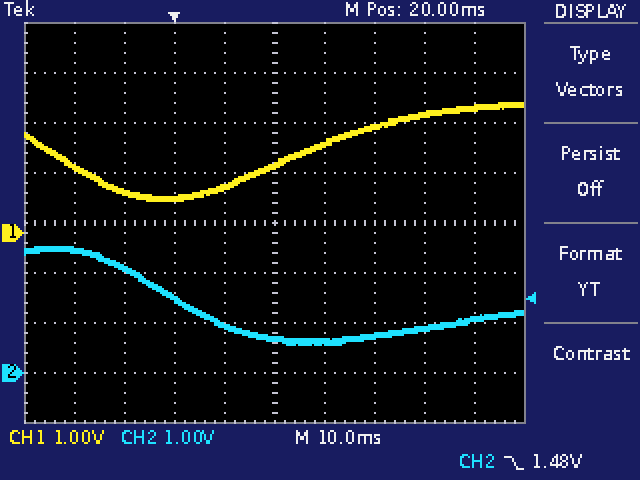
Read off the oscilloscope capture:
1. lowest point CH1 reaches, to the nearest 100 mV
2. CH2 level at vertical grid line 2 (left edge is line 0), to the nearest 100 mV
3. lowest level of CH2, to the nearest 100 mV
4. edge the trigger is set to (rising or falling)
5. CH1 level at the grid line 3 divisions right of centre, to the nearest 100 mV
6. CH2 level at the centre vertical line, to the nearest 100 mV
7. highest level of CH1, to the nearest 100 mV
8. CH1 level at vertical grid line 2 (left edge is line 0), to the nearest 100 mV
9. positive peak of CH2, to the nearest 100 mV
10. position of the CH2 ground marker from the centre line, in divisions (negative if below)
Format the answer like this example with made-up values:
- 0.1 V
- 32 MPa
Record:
- 600 mV
- 2.1 V
- 600 mV
- falling
- 2.4 V
- 700 mV
- 2.6 V
- 800 mV
- 2.5 V
- -3.0 div
